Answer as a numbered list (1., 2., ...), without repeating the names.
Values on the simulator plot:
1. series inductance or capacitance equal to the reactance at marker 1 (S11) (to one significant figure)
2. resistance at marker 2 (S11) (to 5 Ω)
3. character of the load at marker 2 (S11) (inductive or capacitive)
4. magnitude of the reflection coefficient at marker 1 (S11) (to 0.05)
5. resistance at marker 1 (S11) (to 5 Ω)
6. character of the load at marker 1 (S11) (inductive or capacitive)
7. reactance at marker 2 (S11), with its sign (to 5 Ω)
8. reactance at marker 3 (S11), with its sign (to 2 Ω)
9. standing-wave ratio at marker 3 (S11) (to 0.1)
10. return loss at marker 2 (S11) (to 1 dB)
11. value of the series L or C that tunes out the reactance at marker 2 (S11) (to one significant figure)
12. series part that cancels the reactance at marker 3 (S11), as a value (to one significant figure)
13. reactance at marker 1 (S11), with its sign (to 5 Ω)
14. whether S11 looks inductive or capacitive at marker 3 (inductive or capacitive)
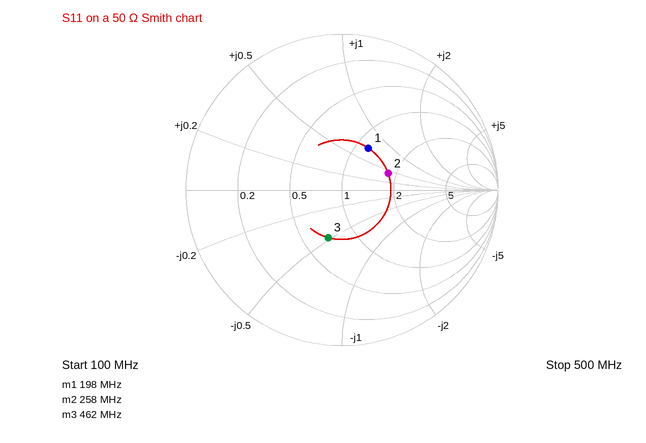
1. 30 nH
2. 90 Ω
3. inductive
4. 0.30
5. 60 Ω
6. inductive
7. +20 Ω
8. -24 Ω
9. 1.9
10. 10 dB
11. 30 pF
12. 8 nH
13. +35 Ω
14. capacitive
